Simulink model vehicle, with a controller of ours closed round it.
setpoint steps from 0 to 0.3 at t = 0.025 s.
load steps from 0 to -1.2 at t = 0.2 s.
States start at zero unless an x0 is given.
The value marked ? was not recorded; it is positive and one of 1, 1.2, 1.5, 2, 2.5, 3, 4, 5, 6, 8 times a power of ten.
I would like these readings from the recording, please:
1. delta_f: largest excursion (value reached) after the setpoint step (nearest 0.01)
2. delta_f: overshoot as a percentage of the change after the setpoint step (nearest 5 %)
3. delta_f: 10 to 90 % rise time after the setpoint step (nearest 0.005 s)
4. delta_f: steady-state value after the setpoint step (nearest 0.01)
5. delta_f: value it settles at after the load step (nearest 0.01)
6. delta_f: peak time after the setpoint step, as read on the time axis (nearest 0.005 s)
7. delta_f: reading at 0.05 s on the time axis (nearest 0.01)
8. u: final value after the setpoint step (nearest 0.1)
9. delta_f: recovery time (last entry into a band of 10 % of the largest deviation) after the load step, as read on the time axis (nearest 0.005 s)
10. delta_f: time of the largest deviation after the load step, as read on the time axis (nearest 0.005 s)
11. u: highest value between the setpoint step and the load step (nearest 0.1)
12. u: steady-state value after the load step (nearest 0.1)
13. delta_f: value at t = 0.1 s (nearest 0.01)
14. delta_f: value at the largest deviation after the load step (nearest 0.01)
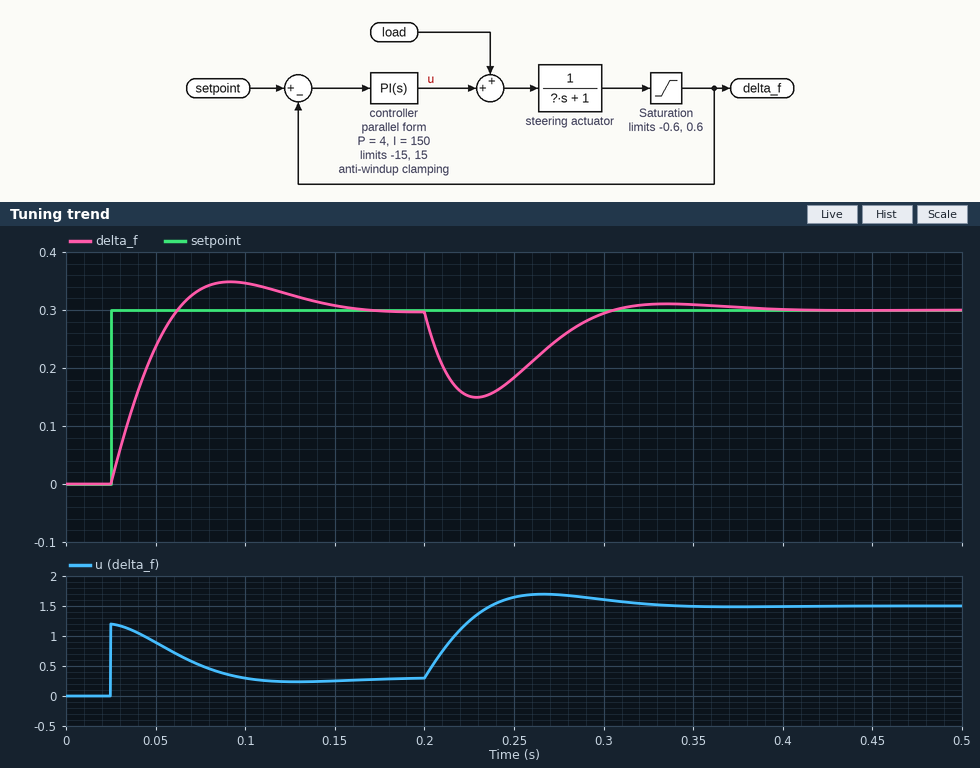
0.35
15 %
0.030 s
0.30
0.30
0.090 s
0.24
0.3
0.295 s
0.230 s
1.2
1.5
0.35
0.15
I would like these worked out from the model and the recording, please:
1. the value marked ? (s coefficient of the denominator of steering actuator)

0.1
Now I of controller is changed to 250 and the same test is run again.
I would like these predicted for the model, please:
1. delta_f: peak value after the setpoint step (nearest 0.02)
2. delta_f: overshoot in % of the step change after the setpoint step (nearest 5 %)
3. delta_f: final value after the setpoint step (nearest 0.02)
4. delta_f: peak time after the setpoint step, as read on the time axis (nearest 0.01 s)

0.38
25 %
0.30
0.08 s
